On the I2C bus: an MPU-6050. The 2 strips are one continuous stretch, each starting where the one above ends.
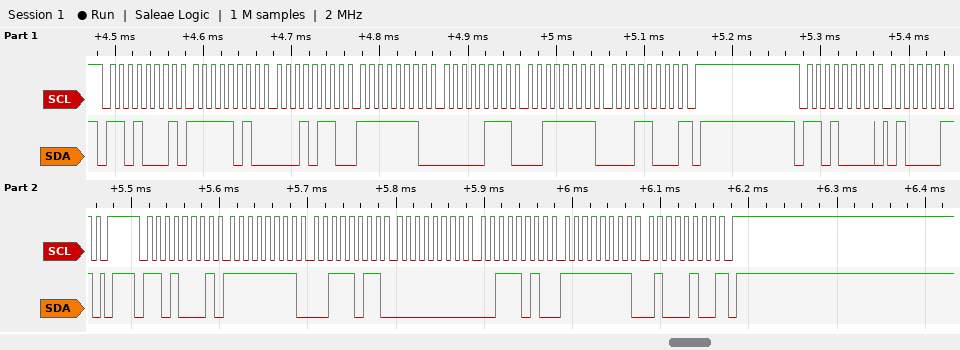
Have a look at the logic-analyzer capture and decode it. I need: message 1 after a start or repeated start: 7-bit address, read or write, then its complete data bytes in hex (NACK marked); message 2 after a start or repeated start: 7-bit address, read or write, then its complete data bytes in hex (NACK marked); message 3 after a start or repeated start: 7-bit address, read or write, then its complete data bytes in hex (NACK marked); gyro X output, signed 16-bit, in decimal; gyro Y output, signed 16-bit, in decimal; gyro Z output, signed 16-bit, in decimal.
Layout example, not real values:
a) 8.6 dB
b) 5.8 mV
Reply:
a) 0x68 read: FA 16 FE 07 3F 18 NACK
b) 0x68 write: 43
c) 0x68 read: FF 3B 00 3A FF 44 NACK
d) -197
e) 58
f) -188
